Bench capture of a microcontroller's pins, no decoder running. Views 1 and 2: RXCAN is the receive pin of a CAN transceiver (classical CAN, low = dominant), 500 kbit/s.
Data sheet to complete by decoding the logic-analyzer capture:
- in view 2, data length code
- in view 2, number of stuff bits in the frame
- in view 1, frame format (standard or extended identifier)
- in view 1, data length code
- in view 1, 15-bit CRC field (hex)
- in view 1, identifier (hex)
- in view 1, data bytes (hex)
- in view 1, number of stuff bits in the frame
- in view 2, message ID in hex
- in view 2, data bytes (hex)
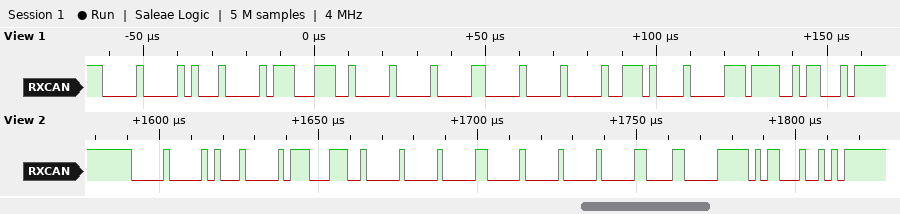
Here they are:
8
12
standard
8
0x5E58
0x001
1C 72 00 02 00 00 E8 41
10
0x001
1C 72 00 02 00 00 10 C1
